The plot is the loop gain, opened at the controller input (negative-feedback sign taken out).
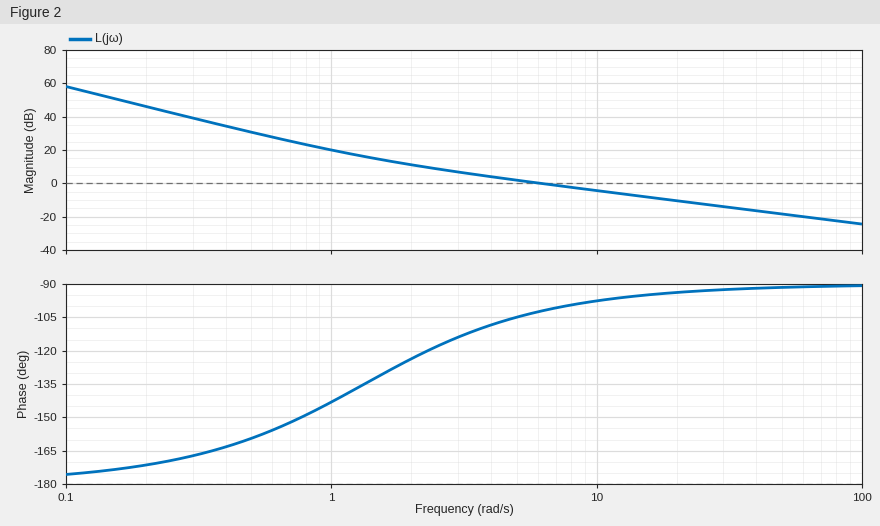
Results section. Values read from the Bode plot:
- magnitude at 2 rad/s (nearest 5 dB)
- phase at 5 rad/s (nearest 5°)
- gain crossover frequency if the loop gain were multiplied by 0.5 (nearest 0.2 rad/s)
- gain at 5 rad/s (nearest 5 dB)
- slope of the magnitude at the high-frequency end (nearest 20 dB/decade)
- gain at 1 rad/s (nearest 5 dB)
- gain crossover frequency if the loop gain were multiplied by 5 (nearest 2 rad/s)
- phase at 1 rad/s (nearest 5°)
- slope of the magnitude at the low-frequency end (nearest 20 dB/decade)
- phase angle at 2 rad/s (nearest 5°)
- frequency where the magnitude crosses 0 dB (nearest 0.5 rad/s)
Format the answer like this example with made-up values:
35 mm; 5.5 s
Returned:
10 dB; -105°; 3.2 rad/s; 0 dB; -20 dB/decade; 20 dB; 30 rad/s; -145°; -40 dB/decade; -125°; 6.0 rad/s
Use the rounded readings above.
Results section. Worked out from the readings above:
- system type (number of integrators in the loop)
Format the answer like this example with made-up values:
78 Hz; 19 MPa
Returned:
2
